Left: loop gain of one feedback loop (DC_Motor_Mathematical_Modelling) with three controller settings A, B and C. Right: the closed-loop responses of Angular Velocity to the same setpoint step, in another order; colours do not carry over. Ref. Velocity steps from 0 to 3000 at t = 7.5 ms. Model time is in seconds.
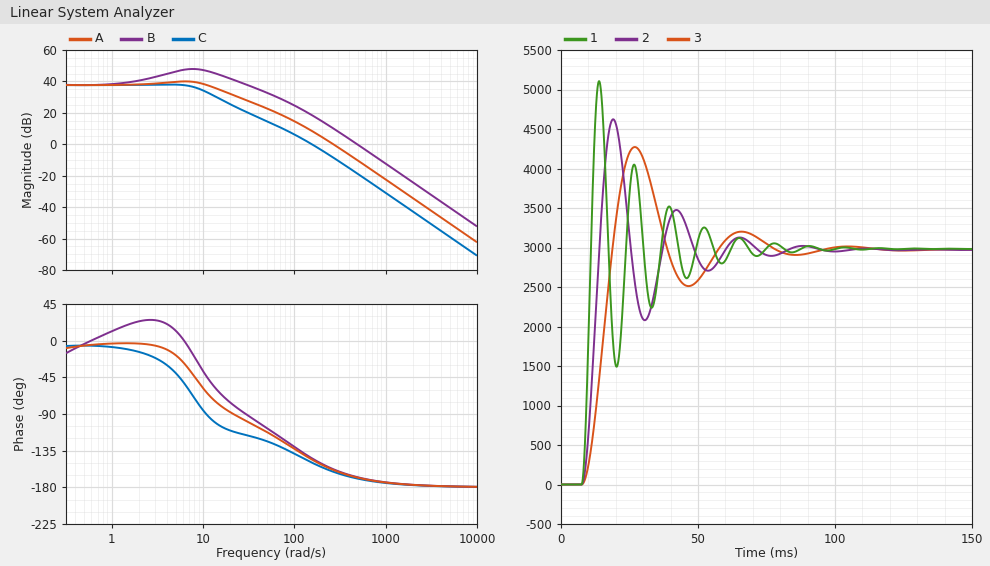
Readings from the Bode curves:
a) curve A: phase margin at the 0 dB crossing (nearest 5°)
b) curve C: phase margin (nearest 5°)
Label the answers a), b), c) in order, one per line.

a) 20°
b) 30°
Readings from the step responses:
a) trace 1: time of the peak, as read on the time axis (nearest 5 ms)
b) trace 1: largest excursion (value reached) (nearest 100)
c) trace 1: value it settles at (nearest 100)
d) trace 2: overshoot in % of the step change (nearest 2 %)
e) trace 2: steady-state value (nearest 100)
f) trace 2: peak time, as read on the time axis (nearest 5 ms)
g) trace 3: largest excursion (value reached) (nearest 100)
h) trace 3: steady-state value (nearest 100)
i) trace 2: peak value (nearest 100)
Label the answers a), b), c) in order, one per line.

a) 15 ms
b) 5100
c) 3000
d) 56 %
e) 3000
f) 20 ms
g) 4300
h) 3000
i) 4600
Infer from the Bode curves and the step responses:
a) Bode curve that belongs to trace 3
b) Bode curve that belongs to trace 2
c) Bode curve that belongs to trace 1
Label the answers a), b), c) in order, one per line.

a) C
b) A
c) B
